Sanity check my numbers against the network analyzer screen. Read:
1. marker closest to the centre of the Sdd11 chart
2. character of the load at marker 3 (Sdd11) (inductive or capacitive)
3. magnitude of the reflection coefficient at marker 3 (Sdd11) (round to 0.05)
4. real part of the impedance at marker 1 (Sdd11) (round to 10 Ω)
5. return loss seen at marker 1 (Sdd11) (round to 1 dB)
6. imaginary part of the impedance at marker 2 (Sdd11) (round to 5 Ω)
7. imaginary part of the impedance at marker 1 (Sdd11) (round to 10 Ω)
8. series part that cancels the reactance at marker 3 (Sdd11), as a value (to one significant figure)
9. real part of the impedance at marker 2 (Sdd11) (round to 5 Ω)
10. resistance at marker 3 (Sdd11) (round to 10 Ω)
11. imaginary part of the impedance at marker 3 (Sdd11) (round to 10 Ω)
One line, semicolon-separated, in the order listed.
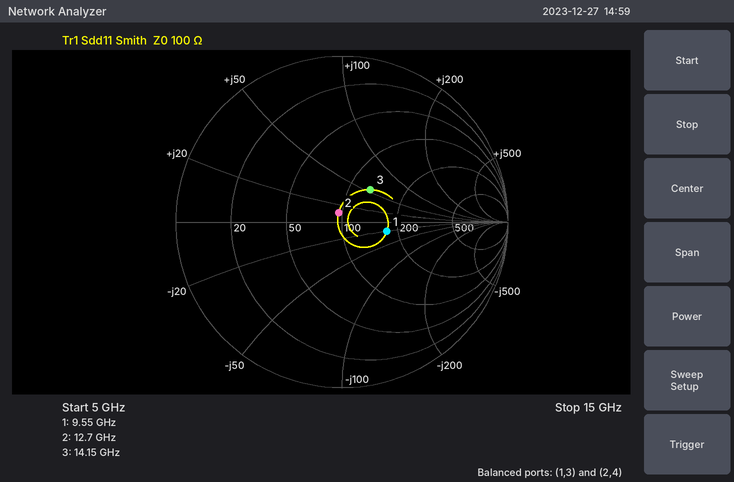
marker 2; inductive; 0.25; 170 Ω; 11 dB; +10 Ω; -20 Ω; 200 fF; 95 Ω; 130 Ω; +50 Ω
